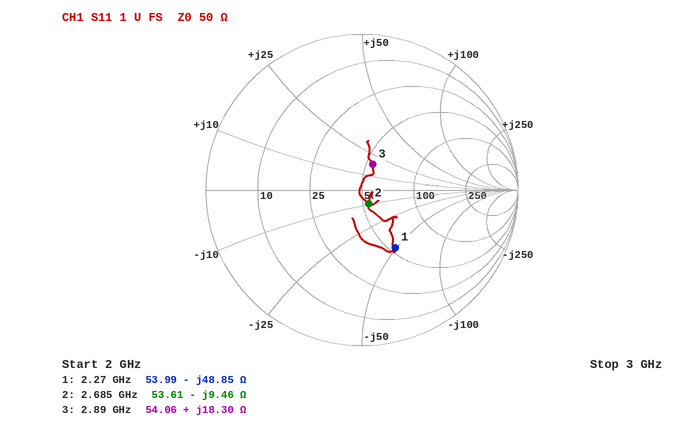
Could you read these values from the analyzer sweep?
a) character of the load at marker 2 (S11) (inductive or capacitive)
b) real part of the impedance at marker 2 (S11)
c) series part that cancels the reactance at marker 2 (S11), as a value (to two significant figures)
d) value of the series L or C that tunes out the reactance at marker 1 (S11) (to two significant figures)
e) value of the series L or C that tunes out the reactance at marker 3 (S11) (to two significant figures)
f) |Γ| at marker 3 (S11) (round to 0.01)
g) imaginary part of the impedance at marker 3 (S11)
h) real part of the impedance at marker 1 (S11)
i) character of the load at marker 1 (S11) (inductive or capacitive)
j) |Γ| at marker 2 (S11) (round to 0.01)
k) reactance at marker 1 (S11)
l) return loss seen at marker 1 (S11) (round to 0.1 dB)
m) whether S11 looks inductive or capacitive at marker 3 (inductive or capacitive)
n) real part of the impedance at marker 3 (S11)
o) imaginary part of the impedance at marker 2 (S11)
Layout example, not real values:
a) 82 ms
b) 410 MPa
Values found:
a) capacitive
b) 53.61 Ω
c) 560 pH
d) 3.4 nH
e) 3.0 pF
f) 0.18
g) +18.30 Ω
h) 53.99 Ω
i) capacitive
j) 0.10
k) -48.85 Ω
l) 7.4 dB
m) inductive
n) 54.06 Ω
o) -9.46 Ω
